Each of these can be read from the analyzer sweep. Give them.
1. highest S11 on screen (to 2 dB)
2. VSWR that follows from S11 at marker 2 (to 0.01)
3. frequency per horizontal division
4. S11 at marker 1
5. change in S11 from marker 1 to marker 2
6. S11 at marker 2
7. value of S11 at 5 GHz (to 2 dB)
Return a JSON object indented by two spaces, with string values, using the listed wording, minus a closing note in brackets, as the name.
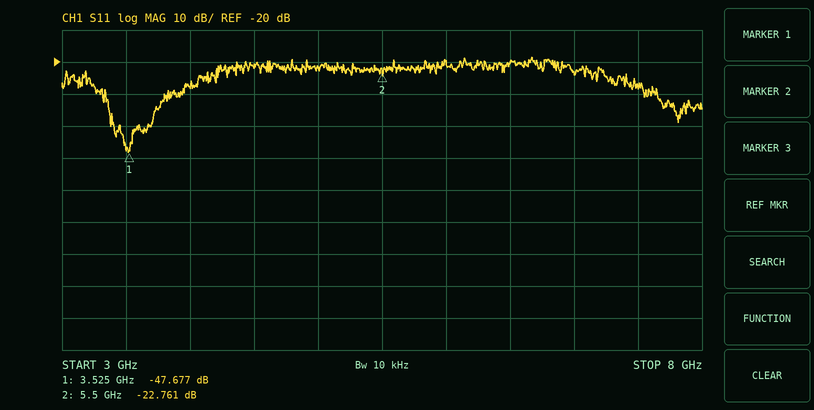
{
  "highest S11 on screen": "-18 dB",
  "VSWR that follows from S11 at marker 2": "1.16",
  "frequency per horizontal division": "500 MHz",
  "S11 at marker 1": "-47.677 dB",
  "change in S11 from marker 1 to marker 2": "24.916 dB",
  "S11 at marker 2": "-22.761 dB",
  "value of S11 at 5 GHz": "-22 dB"
}
